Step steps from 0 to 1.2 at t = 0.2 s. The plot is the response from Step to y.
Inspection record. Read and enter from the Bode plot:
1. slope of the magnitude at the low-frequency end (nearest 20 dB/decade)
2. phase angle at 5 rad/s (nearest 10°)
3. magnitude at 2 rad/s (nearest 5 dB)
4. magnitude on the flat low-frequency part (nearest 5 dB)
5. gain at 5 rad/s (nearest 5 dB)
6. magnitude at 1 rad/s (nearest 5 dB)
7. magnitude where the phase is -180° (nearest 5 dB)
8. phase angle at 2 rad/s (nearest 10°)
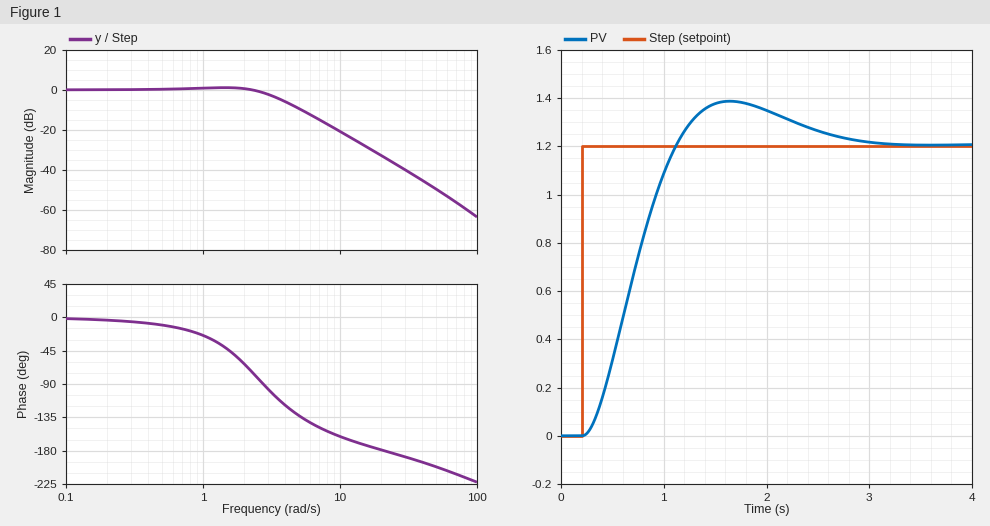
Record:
0 dB/decade
-130°
0 dB
0 dB
-10 dB
0 dB
-35 dB
-60°
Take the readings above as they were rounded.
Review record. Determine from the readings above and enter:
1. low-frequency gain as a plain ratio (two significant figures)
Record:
1.0
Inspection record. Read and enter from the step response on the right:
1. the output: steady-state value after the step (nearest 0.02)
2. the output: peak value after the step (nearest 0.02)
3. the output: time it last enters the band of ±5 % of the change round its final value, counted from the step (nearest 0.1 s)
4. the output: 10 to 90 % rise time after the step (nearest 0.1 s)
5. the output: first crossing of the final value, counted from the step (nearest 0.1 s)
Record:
1.20
1.38
2.3 s
0.6 s
0.9 s
